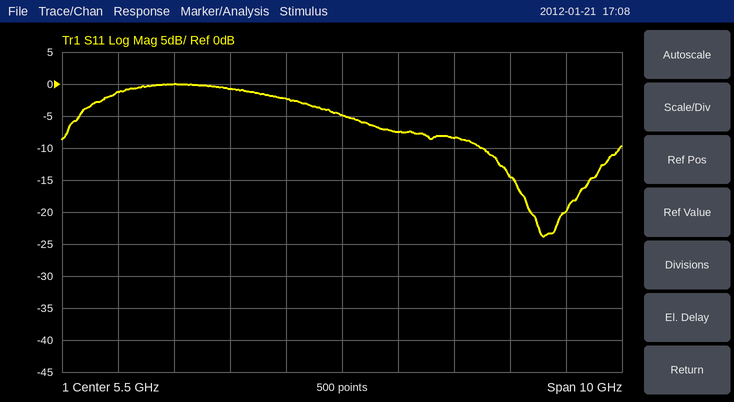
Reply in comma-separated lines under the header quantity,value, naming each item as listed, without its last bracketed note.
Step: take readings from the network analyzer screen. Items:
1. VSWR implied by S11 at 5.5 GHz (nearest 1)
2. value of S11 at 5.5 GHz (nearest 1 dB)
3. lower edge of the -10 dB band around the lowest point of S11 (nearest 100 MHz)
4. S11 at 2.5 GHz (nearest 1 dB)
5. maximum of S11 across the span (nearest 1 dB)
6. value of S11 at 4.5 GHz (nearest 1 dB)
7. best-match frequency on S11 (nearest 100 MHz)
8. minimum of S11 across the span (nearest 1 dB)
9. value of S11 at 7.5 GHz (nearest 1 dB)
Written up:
quantity,value
VSWR implied by S11 at 5.5 GHz,4
value of S11 at 5.5 GHz,-5 dB
lower edge of the -10 dB band around the lowest point of S11,8.0 GHz
S11 at 2.5 GHz,0 dB
maximum of S11 across the span,0 dB
value of S11 at 4.5 GHz,-2 dB
best-match frequency on S11,9.1 GHz
minimum of S11 across the span,-24 dB
value of S11 at 7.5 GHz,-8 dB
